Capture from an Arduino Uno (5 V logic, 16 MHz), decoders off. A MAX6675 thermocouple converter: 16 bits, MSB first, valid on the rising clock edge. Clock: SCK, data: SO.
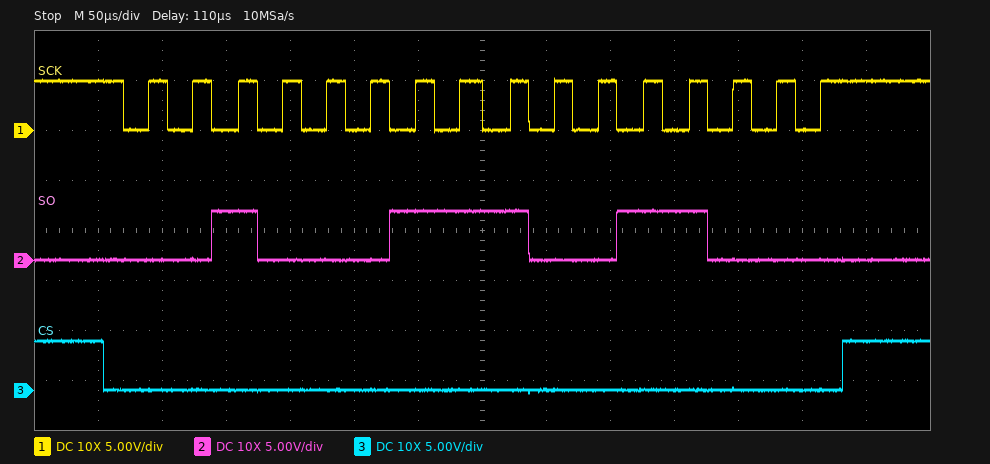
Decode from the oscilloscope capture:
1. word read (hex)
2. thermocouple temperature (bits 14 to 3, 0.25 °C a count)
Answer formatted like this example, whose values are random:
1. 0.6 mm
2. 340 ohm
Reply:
1. 0x2398
2. 284.75 °C
